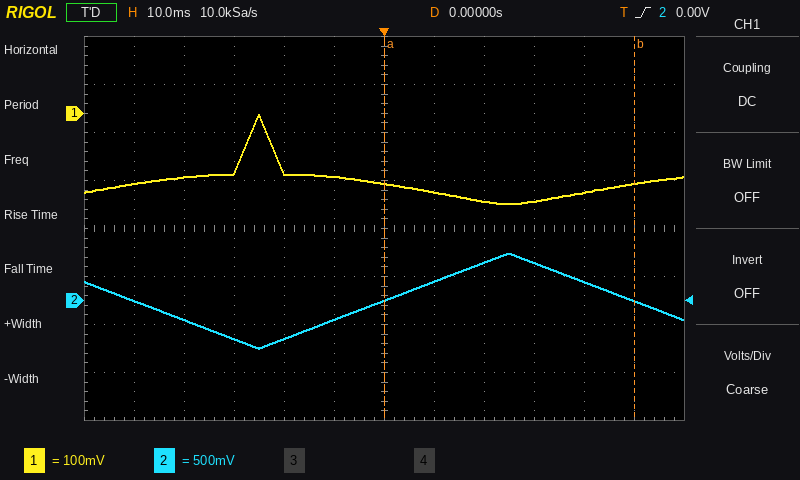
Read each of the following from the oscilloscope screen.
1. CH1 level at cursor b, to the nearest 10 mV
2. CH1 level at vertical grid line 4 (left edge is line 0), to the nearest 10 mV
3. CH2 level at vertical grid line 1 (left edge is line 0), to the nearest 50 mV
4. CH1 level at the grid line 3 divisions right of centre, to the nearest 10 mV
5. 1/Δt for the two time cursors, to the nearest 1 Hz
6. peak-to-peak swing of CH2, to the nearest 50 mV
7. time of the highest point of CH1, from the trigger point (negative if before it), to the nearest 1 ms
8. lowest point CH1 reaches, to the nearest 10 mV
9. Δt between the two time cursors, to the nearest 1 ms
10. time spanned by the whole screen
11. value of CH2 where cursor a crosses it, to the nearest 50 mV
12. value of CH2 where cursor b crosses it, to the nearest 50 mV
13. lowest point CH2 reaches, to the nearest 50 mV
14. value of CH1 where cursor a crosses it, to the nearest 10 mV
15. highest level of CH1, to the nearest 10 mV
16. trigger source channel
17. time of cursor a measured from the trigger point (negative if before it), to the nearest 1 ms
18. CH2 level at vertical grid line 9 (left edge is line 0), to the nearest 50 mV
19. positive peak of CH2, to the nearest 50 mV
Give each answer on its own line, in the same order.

-150 mV
-120 mV
0 mV
-180 mV
20 Hz
1.00 V
-25 ms
-190 mV
50 ms
120 ms
0 mV
0 mV
-500 mV
-150 mV
0 mV
CH2
0 ms
400 mV
500 mV
